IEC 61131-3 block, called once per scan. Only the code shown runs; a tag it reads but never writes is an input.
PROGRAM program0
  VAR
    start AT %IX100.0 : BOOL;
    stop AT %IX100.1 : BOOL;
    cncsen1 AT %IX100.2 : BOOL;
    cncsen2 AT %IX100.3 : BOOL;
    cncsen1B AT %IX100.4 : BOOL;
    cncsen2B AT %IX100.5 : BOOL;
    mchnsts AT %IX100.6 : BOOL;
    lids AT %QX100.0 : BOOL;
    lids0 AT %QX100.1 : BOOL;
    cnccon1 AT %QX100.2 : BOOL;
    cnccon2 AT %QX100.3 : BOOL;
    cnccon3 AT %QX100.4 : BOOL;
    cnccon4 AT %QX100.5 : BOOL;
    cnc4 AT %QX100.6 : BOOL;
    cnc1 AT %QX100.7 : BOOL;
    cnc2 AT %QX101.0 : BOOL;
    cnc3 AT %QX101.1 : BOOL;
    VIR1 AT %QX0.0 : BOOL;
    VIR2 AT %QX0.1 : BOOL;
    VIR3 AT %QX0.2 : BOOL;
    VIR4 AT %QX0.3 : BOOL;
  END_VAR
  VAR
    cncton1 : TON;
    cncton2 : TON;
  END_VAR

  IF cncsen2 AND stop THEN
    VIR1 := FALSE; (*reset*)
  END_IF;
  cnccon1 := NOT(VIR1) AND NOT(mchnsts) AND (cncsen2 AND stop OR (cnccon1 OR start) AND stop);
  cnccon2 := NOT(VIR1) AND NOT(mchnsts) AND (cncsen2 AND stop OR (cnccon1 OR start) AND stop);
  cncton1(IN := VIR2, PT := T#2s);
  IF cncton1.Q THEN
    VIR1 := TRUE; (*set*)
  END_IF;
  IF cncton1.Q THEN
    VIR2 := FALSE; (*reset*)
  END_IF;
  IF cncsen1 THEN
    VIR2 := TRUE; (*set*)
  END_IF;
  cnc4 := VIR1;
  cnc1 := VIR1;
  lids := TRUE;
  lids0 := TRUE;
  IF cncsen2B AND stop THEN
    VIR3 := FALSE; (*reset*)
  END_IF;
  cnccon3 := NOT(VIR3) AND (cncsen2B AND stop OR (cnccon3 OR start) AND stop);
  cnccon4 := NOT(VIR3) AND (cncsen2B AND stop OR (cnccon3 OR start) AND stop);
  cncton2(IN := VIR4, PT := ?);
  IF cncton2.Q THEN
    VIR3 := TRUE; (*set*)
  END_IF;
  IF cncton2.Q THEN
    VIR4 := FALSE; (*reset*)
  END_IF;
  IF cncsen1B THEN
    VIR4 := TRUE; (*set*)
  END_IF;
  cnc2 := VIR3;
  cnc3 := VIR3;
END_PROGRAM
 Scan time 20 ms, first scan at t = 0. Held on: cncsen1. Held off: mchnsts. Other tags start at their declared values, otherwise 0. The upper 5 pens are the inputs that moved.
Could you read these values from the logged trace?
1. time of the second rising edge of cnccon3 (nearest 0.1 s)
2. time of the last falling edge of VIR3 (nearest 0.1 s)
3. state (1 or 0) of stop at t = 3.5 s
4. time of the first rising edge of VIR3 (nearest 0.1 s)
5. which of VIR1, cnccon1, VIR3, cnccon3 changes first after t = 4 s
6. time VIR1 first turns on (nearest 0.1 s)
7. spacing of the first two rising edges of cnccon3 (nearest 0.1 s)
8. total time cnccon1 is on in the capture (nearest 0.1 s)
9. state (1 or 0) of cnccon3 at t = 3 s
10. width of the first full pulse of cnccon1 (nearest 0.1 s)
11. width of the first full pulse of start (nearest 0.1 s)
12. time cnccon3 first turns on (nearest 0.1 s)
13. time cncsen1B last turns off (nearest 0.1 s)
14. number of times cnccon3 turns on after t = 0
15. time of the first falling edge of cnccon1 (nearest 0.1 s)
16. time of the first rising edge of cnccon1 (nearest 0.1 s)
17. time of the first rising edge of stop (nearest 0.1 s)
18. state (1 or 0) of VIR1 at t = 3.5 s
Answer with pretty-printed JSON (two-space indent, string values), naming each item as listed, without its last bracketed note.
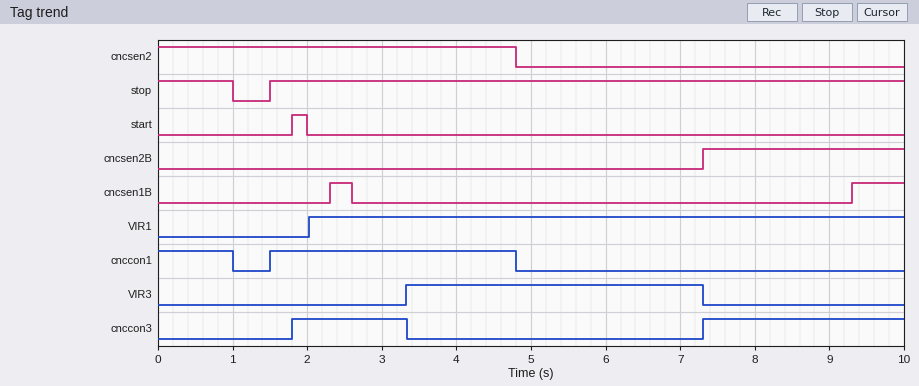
{
  "time of the second rising edge of cnccon3": "7.3 s",
  "time of the last falling edge of VIR3": "7.3 s",
  "state (1 or 0) of stop at t = 3.5 s": "1",
  "time of the first rising edge of VIR3": "3.3 s",
  "which of VIR1, cnccon1, VIR3, cnccon3 changes first after t = 4 s": "cnccon1",
  "time VIR1 first turns on": "2.0 s",
  "spacing of the first two rising edges of cnccon3": "5.5 s",
  "total time cnccon1 is on in the capture": "4.3 s",
  "state (1 or 0) of cnccon3 at t = 3 s": "1",
  "width of the first full pulse of cnccon1": "3.3 s",
  "width of the first full pulse of start": "0.2 s",
  "time cnccon3 first turns on": "1.8 s",
  "time cncsen1B last turns off": "2.6 s",
  "number of times cnccon3 turns on after t = 0": "2",
  "time of the first falling edge of cnccon1": "1.0 s",
  "time of the first rising edge of cnccon1": "1.5 s",
  "time of the first rising edge of stop": "1.5 s",
  "state (1 or 0) of VIR1 at t = 3.5 s": "1"
}
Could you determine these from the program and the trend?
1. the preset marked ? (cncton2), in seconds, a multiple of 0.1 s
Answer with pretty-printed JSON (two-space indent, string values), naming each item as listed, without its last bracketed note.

{
  "the preset marked ? (cncton2), in seconds, a multiple of 0.1 s": "1.0 s"
}
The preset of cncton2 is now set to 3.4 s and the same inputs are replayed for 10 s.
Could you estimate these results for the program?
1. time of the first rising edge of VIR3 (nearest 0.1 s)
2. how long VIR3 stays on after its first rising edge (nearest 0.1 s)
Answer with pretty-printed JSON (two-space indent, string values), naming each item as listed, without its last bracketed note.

{
  "time of the first rising edge of VIR3": "5.7 s",
  "how long VIR3 stays on after its first rising edge": "1.6 s"
}
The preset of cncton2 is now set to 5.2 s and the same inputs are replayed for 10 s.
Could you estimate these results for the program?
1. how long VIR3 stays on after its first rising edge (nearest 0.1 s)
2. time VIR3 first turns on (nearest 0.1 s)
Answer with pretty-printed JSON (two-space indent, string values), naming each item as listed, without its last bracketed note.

{
  "how long VIR3 stays on after its first rising edge": "0.0 s",
  "time VIR3 first turns on": "7.5 s"
}
